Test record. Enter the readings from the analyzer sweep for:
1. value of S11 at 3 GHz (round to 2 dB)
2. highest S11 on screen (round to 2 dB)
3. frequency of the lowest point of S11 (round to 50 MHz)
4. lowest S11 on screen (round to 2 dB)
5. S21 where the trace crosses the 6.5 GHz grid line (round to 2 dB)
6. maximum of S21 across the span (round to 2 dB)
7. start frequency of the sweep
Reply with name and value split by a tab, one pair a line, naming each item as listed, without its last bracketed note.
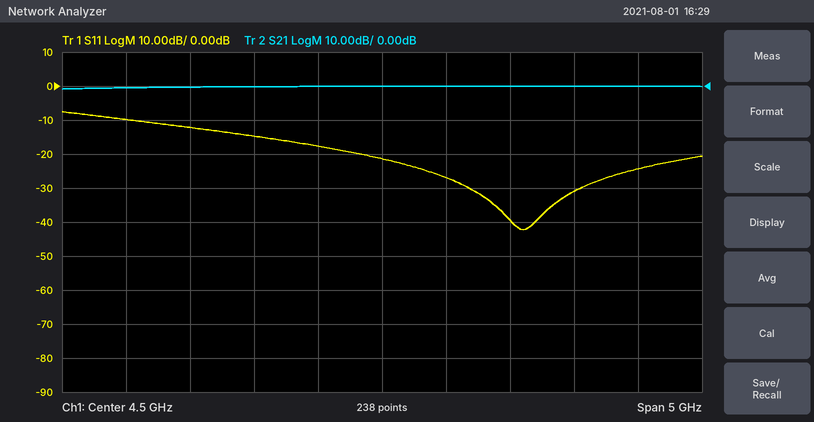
value of S11 at 3 GHz	-12 dB
highest S11 on screen	-8 dB
frequency of the lowest point of S11	5.60 GHz
lowest S11 on screen	-42 dB
S21 where the trace crosses the 6.5 GHz grid line	0 dB
maximum of S21 across the span	0 dB
start frequency of the sweep	2 GHz
